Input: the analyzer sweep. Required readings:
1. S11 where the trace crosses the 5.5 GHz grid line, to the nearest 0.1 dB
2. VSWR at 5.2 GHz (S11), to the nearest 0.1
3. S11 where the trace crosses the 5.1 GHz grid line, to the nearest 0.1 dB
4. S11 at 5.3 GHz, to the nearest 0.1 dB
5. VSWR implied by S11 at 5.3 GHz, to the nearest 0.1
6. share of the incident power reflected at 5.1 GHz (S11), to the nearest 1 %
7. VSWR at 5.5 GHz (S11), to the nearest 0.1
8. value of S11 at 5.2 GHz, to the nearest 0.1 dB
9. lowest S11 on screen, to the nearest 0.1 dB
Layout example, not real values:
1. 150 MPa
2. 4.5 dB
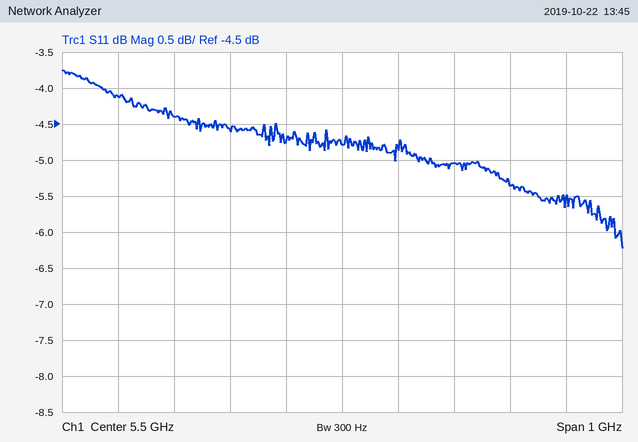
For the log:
1. -4.8 dB
2. 4.0
3. -4.1 dB
4. -4.6 dB
5. 3.9
6. 39 %
7. 3.7
8. -4.4 dB
9. -6.2 dB
